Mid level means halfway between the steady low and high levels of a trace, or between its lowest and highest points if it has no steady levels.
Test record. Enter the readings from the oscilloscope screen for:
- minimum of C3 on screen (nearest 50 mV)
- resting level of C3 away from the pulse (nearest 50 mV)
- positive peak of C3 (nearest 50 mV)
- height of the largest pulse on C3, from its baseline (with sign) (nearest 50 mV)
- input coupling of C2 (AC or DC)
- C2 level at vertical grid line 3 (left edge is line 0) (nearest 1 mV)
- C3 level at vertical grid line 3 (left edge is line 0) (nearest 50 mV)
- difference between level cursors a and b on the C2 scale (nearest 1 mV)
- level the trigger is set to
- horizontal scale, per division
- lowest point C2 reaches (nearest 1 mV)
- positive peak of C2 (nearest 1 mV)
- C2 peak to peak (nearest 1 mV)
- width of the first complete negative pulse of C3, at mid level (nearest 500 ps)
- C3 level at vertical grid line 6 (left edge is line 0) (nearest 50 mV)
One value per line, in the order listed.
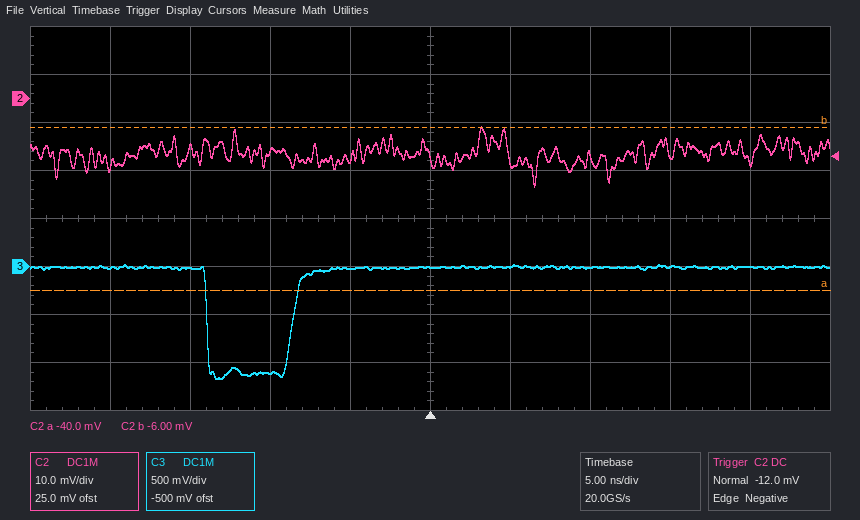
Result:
-1.15 V
0 mV
0 mV
-1.15 V
DC
-11 mV
-1.10 V
34 mV
-12.0 mV
5 ns
-18 mV
-6 mV
12 mV
5.5 ns
0 mV
